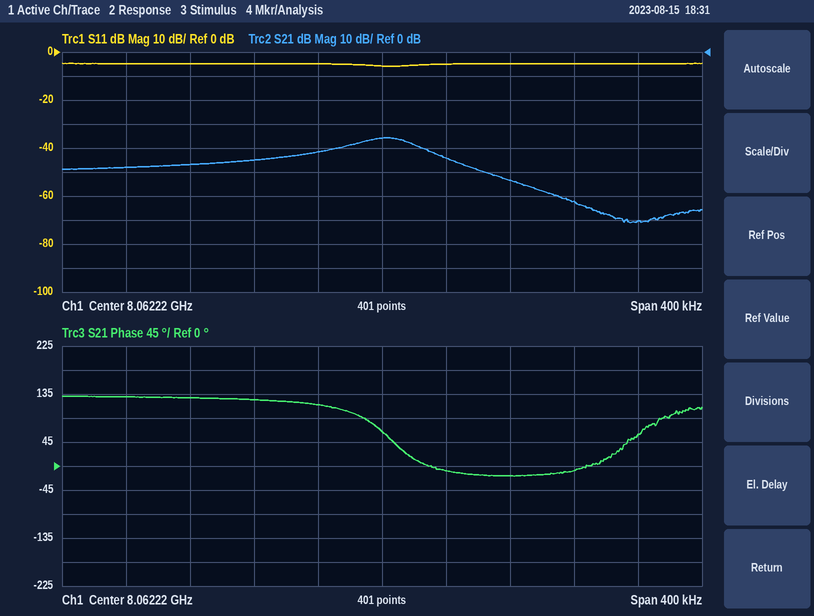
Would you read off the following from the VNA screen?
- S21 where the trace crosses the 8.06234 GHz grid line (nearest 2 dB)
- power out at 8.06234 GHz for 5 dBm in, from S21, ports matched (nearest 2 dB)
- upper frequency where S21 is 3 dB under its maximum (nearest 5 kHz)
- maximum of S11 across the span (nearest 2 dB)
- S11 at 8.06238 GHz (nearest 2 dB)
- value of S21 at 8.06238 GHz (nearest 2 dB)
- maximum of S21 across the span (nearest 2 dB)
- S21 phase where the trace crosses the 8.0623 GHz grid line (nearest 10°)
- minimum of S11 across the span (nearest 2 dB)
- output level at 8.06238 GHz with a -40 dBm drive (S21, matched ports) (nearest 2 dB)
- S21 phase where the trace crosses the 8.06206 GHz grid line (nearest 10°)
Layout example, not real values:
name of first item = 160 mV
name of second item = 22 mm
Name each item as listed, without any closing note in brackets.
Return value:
S21 where the trace crosses the 8.06234 GHz grid line = -62 dB
power out at 8.06234 GHz for 5 dBm in, from S21, ports matched = -58 dBm
upper frequency where S21 is 3 dB under its maximum = 8.062240 GHz
maximum of S11 across the span = -4 dB
S11 at 8.06238 GHz = -4 dB
value of S21 at 8.06238 GHz = -70 dB
maximum of S21 across the span = -36 dB
S21 phase where the trace crosses the 8.0623 GHz grid line = -20°
minimum of S11 across the span = -6 dB
output level at 8.06238 GHz with a -40 dBm drive (S21, matched ports) = -110 dBm
S21 phase where the trace crosses the 8.06206 GHz grid line = 130°
